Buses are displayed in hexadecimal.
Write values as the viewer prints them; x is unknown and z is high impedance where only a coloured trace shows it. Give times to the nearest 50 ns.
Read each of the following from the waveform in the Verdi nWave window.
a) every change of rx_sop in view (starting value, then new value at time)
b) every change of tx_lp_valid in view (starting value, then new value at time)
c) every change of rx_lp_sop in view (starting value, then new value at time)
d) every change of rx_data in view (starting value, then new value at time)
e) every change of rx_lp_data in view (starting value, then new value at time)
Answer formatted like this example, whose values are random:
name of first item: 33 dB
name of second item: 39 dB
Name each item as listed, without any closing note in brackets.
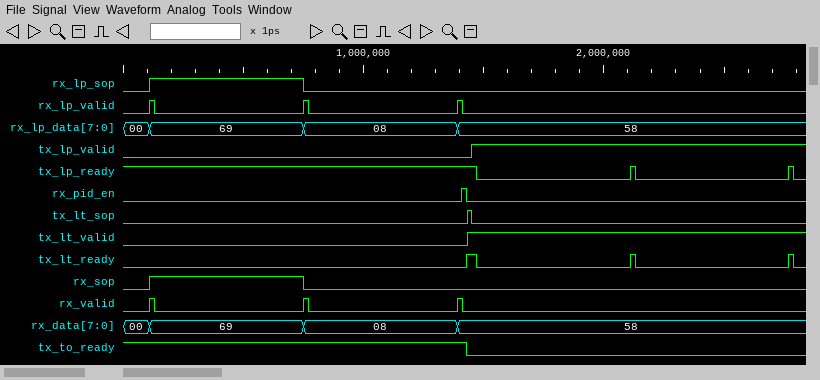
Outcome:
every change of rx_sop in view: 0, 1 at 100 ns, 0 at 750 ns
every change of tx_lp_valid in view: 0, 1 at 1450 ns
every change of rx_lp_sop in view: 0, 1 at 100 ns, 0 at 750 ns
every change of rx_data in view: 00, 69 at 100 ns, 08 at 750 ns, 58 at 1400 ns
every change of rx_lp_data in view: 00, 69 at 100 ns, 08 at 750 ns, 58 at 1400 ns
